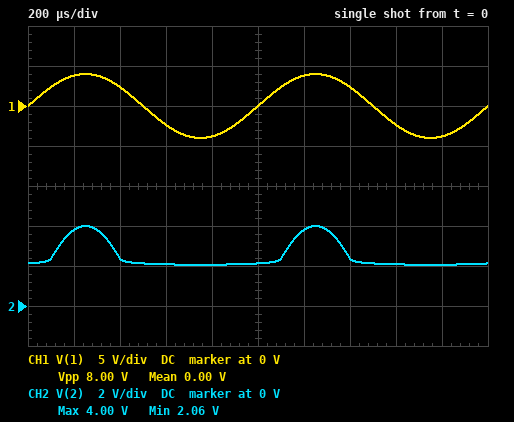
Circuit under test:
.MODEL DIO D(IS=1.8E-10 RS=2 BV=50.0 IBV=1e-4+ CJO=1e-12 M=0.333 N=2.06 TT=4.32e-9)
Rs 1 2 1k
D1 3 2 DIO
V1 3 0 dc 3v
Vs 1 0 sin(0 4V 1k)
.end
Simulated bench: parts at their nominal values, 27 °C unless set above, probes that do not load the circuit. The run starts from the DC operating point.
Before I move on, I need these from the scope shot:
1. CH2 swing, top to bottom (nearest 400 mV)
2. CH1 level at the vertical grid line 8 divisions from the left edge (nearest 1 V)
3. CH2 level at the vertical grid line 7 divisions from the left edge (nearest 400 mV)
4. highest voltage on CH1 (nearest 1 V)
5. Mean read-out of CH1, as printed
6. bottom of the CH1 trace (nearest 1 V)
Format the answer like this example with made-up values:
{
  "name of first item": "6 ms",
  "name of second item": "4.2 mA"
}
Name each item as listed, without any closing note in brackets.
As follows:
{
  "CH2 swing, top to bottom": "2.0 V",
  "CH1 level at the vertical grid line 8 divisions from the left edge": "-2 V",
  "CH2 level at the vertical grid line 7 divisions from the left edge": "2.4 V",
  "highest voltage on CH1": "4 V",
  "Mean read-out of CH1, as printed": "0.00 V",
  "bottom of the CH1 trace": "-4 V"
}
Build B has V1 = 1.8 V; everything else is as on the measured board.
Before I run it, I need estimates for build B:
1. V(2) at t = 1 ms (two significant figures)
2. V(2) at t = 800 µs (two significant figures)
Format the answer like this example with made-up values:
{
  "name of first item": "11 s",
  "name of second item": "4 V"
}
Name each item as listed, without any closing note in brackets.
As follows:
{
  "V(2) at t = 1 ms": "970 mV",
  "V(2) at t = 800 µs": "880 mV"
}
